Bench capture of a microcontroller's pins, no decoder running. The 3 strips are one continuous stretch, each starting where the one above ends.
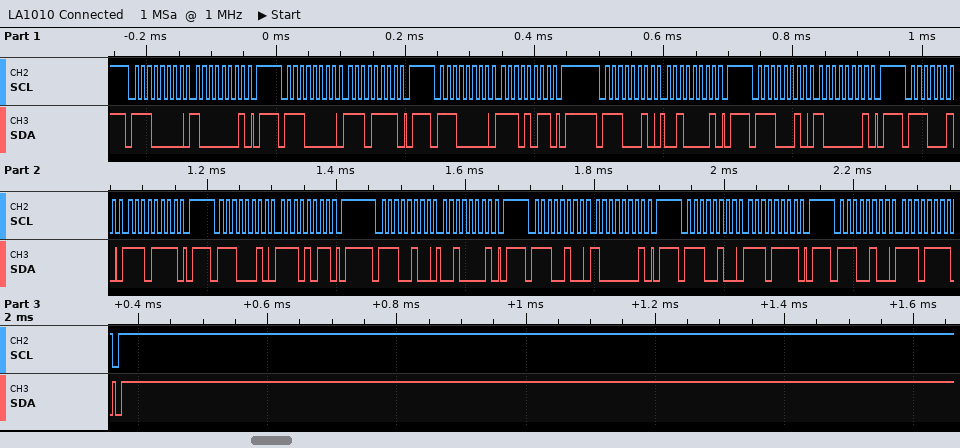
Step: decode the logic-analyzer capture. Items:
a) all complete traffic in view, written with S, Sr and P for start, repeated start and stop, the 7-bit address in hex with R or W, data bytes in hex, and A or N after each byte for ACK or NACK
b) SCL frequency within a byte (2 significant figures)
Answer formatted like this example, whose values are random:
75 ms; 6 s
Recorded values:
S 70W A 81 A P S 70W A EF A P S 70W A EB A P S 71W A 21 A P S 71W A 81 A P S 71W A EF A P S 71W A EB A P S 72W A 21 A P S 72W A 81 A P S 72W A EF A P S 72W A EF A P; 100 kHz
